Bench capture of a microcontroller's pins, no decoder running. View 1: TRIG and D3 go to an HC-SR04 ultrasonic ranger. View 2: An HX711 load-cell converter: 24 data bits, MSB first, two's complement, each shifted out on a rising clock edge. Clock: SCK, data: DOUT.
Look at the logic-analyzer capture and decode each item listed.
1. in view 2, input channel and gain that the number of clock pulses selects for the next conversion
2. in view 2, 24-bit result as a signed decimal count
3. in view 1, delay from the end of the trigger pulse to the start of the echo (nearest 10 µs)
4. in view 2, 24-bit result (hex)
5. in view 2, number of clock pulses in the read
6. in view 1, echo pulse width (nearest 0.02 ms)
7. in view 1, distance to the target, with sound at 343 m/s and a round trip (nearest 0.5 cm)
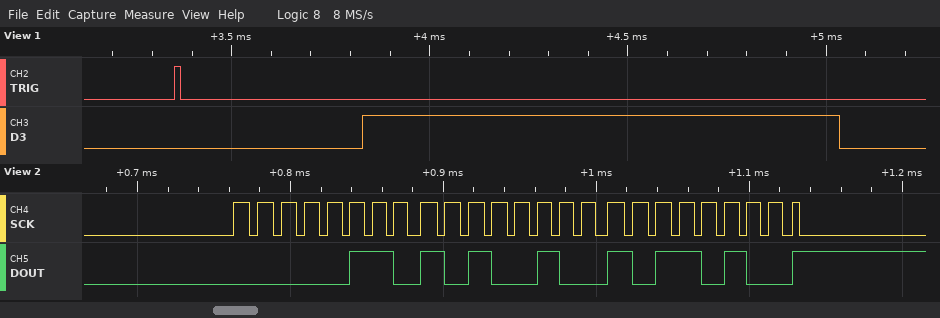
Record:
channel A, gain 128
435380
460 µs
0x06A4B4
25
1.20 ms
20.5 cm
